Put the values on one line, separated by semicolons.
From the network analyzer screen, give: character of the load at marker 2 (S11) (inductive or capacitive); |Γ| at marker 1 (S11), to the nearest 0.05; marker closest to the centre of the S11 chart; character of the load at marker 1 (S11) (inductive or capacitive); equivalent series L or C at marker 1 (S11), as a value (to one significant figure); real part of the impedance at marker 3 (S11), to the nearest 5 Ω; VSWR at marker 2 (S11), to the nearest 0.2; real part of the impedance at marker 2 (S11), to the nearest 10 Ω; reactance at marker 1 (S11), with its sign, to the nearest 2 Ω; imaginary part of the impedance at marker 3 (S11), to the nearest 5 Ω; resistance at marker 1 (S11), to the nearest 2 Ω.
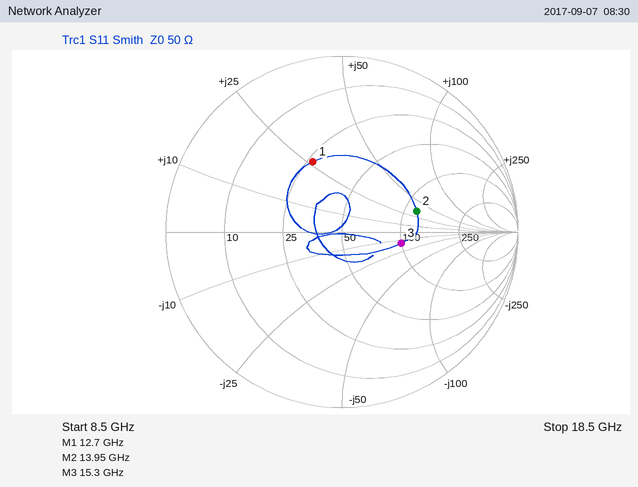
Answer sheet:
inductive; 0.45; marker 3; inductive; 300 pH; 100 Ω; 2.6; 120 Ω; +26 Ω; -15 Ω; 26 Ω
